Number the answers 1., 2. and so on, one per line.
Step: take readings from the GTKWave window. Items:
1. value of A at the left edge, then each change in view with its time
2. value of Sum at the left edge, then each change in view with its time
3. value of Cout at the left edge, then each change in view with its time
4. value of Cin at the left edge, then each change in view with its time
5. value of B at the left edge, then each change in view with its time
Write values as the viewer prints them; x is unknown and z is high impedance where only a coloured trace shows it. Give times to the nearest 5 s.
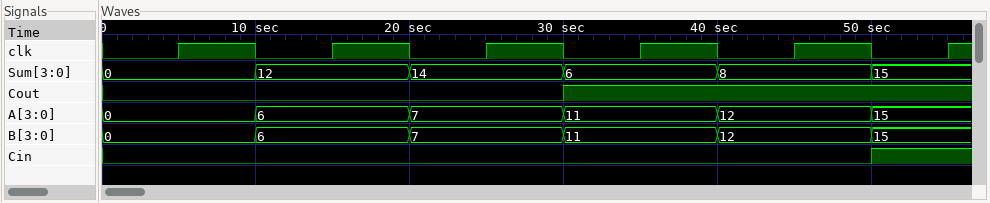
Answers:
1. 0, 6 at 10 s, 7 at 20 s, 11 at 30 s, 12 at 40 s, 15 at 50 s
2. 0, 12 at 10 s, 14 at 20 s, 6 at 30 s, 8 at 40 s, 15 at 50 s
3. 0, 1 at 30 s
4. 0, 1 at 50 s
5. 0, 6 at 10 s, 7 at 20 s, 11 at 30 s, 12 at 40 s, 15 at 50 s
